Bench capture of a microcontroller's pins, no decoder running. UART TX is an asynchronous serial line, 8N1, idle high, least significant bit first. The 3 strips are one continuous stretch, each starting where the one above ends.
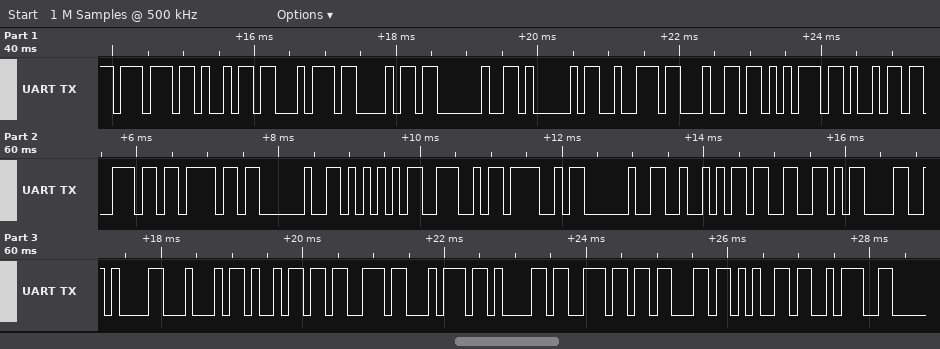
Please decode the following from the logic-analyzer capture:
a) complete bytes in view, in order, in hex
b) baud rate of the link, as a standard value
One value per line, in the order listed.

77 69 74 68 20 41 72 64 75 69 6E 6F 20 55 4E 4F 20 52 33 0D 0A 44 69 73 74 61 6E 63 65 3A
9600 baud
